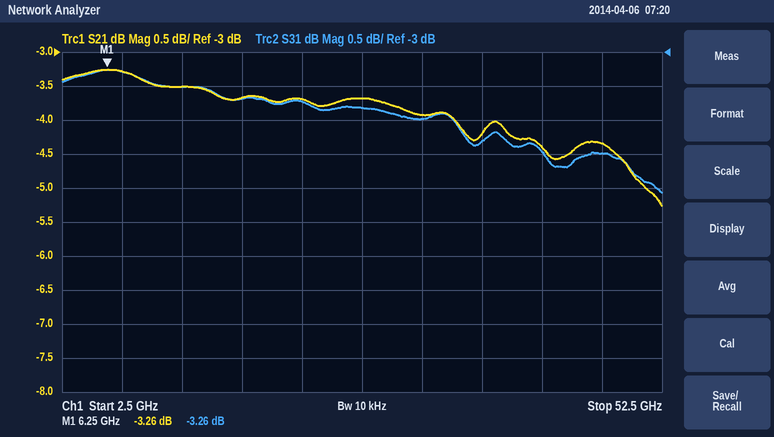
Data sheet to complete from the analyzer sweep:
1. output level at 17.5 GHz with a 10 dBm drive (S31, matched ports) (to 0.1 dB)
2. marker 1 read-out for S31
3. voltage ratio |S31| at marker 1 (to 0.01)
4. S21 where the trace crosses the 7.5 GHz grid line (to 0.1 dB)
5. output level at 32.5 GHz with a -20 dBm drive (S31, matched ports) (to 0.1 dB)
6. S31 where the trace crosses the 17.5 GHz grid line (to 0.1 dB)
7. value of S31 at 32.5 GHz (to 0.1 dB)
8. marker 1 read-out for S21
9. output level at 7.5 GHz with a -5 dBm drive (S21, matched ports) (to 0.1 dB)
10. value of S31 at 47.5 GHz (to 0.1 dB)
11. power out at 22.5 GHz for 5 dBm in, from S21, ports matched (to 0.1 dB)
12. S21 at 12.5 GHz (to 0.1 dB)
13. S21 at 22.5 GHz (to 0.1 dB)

6.3 dBm
-3.26 dB
0.69
-3.3 dB
-24.0 dBm
-3.7 dB
-4.0 dB
-3.26 dB
-8.3 dBm
-4.5 dB
1.3 dBm
-3.5 dB
-3.7 dB
